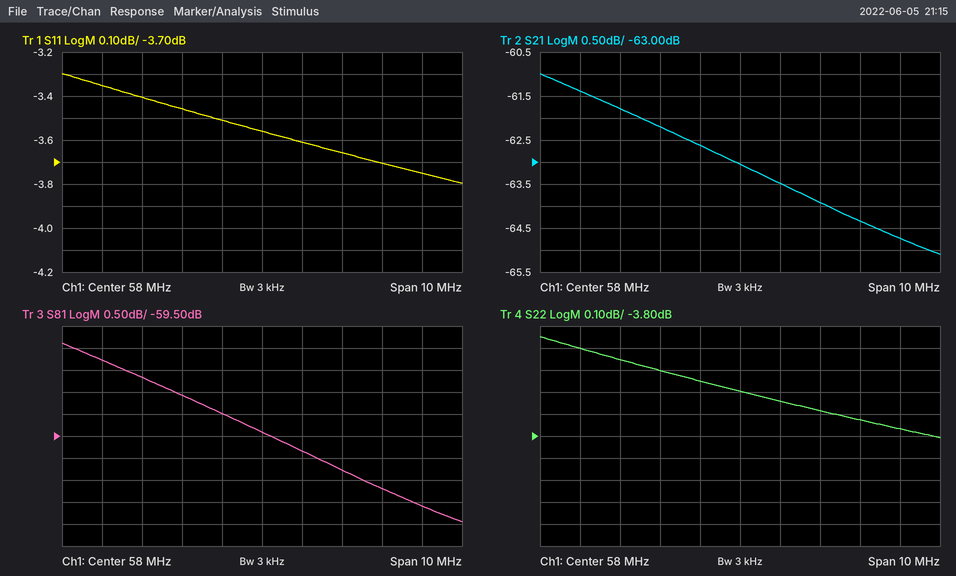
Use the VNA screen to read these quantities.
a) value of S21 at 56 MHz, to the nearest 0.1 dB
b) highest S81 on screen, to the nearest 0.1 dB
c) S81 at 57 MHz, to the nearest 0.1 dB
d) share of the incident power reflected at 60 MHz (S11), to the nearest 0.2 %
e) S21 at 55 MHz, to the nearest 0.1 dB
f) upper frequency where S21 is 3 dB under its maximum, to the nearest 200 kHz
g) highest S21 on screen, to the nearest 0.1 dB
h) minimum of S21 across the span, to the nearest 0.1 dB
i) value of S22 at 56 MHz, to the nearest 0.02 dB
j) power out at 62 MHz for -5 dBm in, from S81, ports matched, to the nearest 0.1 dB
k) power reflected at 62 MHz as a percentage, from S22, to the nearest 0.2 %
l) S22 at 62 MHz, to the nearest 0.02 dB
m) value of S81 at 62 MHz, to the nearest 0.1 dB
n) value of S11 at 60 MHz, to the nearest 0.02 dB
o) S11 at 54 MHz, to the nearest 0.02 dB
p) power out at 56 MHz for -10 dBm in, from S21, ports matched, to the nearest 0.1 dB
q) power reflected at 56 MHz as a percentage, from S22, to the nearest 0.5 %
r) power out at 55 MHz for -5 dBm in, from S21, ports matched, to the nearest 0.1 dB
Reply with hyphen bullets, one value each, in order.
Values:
- -62.2 dB
- -57.4 dB
- -59.0 dB
- 43.0 %
- -61.8 dB
- 60.2 MHz
- -61.0 dB
- -65.1 dB
- -3.50 dB
- -66.1 dBm
- 42.0 %
- -3.76 dB
- -61.1 dB
- -3.66 dB
- -3.36 dB
- -72.2 dBm
- 44.5 %
- -66.8 dBm
